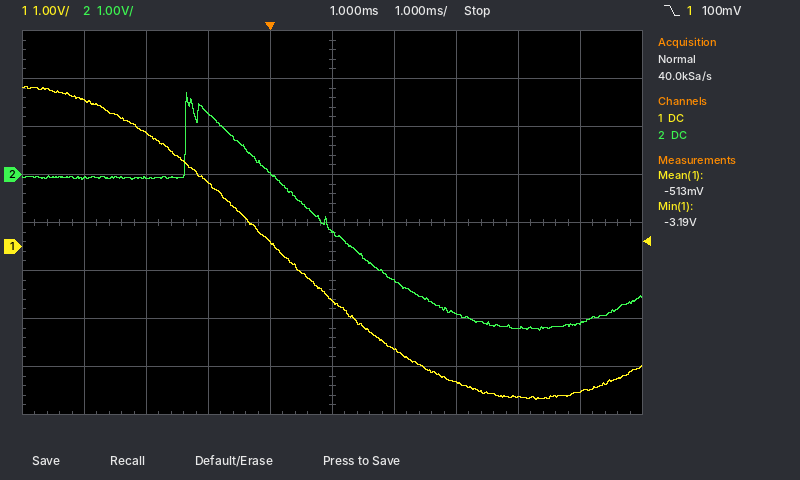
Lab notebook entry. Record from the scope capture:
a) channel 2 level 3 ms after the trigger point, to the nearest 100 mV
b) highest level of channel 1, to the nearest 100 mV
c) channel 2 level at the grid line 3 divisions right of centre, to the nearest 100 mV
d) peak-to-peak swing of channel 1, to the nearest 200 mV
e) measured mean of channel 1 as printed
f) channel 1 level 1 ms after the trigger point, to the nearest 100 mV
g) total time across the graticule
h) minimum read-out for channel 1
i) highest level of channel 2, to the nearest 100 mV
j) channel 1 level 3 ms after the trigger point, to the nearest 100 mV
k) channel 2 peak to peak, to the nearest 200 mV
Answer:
-2.9 V
3.3 V
-3.2 V
6.6 V
-513 mV
-1.1 V
10 ms
-3.19 V
1.7 V
-2.8 V
5.0 V
